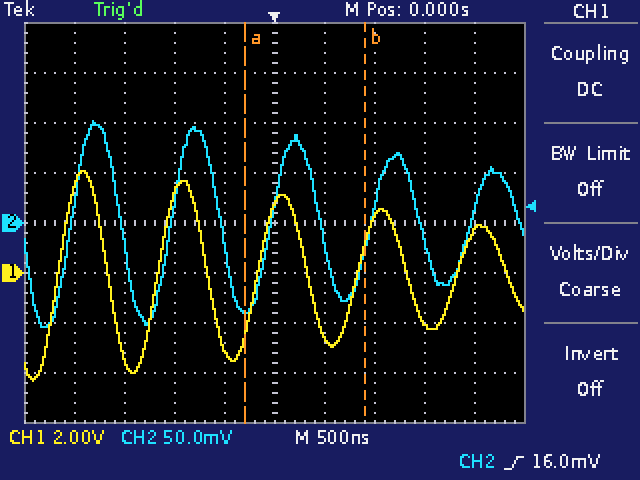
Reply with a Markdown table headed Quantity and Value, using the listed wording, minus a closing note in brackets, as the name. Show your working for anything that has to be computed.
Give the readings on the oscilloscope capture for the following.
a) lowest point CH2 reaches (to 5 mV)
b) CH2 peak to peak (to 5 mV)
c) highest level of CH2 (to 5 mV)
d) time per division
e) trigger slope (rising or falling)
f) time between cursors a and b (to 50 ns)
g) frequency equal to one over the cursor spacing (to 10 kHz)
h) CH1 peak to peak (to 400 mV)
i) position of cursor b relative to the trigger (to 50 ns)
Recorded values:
| Quantity | Value |
|---|---|
| lowest point CH2 reaches | -105 mV |
| CH2 peak to peak | 100 mV − (-105 mV) = 205 mV |
| highest level of CH2 | 100 mV |
| time per division | 500 ns |
| trigger slope | rising |
| time between cursors a and b | 1.20 µs |
| frequency equal to one over the cursor spacing | 1 / 1.20 µs ≈ 830 kHz |
| CH1 peak to peak | 8.4 V |
| position of cursor b relative to the trigger | +900 ns |
